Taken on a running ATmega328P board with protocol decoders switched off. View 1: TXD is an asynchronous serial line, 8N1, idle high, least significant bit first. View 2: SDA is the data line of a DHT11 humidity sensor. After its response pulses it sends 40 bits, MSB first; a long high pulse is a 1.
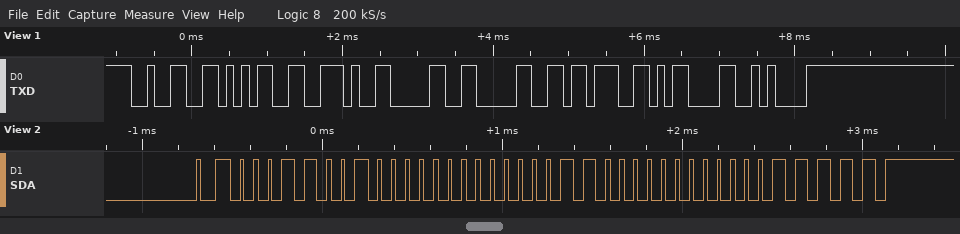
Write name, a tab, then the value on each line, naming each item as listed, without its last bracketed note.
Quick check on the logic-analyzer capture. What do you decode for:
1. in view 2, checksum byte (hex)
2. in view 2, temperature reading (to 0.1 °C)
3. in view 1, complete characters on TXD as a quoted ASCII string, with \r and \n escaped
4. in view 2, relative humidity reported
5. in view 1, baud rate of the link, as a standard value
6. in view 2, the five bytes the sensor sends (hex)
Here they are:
in view 2, checksum byte	0x1F
in view 2, temperature reading	6.0 °C
in view 1, complete characters on TXD as a quoted ASCII string, with \r and \n escaped	"25.00;\r\n"
in view 2, relative humidity reported	25 %
in view 1, baud rate of the link, as a standard value	9600 baud
in view 2, the five bytes the sensor sends	19 00 06 00 1F
